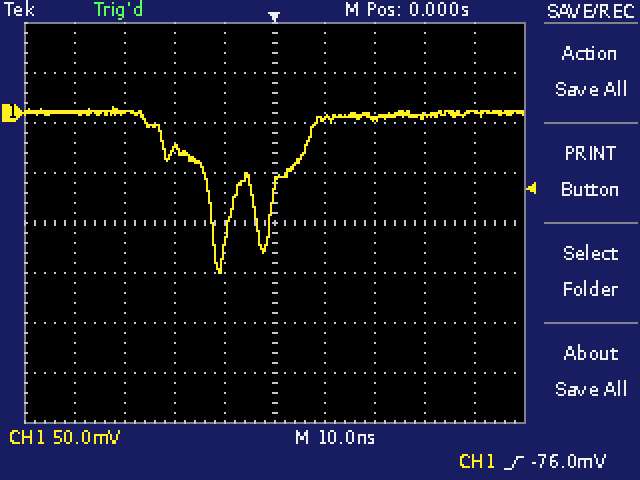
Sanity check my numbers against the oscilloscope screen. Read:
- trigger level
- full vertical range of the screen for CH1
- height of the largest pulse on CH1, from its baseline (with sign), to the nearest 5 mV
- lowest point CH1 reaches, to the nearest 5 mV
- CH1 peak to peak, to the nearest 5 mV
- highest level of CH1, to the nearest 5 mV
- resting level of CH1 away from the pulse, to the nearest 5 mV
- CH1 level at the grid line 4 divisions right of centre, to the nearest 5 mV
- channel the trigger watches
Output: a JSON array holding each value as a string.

["-76.0 mV", "400 mV", "-160 mV", "-160 mV", "165 mV", "5 mV", "0 mV", "0 mV", "CH1"]
